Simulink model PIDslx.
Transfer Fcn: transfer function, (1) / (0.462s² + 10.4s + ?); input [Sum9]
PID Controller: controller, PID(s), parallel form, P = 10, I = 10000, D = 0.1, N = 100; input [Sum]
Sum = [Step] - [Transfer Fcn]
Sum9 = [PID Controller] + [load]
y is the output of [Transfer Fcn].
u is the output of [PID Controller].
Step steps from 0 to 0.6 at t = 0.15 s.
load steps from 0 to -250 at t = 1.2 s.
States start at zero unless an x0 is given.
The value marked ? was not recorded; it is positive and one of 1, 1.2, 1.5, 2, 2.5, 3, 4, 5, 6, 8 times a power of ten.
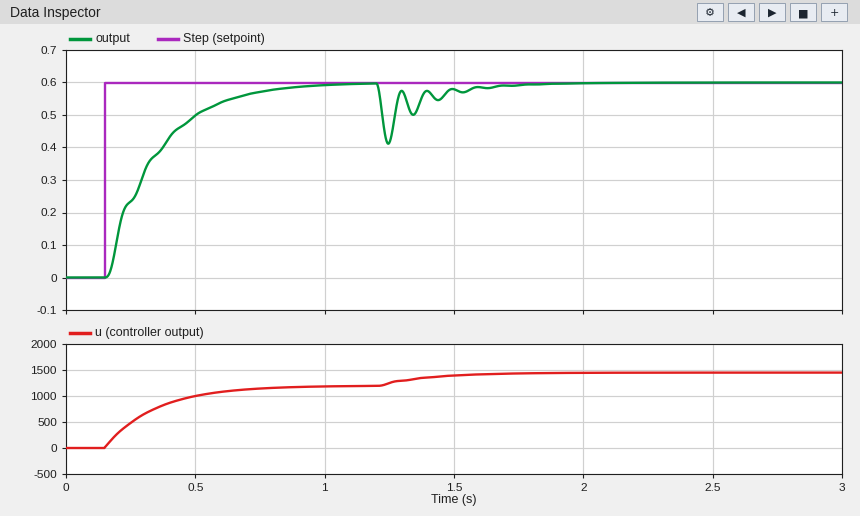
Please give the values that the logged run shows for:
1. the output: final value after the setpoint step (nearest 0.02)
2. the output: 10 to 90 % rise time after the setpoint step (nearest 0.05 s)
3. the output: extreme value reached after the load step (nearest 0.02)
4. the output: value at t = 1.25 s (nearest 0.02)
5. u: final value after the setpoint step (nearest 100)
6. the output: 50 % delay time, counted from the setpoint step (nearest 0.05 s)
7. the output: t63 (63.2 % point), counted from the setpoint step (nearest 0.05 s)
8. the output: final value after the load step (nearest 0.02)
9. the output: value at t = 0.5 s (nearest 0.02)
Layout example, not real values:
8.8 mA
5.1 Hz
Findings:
0.60
0.40 s
0.42
0.42
1200
0.15 s
0.20 s
0.60
0.50
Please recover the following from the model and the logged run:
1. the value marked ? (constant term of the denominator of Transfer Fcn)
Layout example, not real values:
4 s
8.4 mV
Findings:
2000
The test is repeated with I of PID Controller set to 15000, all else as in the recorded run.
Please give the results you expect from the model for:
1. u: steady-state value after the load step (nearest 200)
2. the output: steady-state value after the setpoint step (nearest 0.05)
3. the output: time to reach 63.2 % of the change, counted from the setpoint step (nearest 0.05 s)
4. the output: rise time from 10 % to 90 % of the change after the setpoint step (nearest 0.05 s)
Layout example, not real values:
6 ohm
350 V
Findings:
1400
0.60
0.15 s
0.30 s
